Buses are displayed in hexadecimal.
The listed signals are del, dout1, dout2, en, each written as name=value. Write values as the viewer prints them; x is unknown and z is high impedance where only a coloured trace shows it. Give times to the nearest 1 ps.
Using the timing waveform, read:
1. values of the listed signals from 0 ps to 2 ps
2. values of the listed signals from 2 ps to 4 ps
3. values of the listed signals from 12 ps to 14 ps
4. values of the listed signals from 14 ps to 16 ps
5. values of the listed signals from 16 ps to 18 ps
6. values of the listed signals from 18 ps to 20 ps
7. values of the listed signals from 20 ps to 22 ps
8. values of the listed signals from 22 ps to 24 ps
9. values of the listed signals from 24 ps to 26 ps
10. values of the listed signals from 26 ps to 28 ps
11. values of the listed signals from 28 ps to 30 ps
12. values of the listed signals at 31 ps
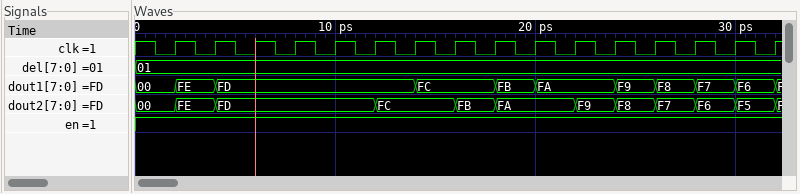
del=01, dout1=00, dout2=00, en=1
del=01, dout1=FE, dout2=FE, en=1
del=01, dout1=FD, dout2=FC, en=1
del=01, dout1=FC, dout2=FC, en=1
del=01, dout1=FC, dout2=FB, en=1
del=01, dout1=FB, dout2=FA, en=1
del=01, dout1=FA, dout2=FA, en=1
del=01, dout1=FA, dout2=F9, en=1
del=01, dout1=F9, dout2=F8, en=1
del=01, dout1=F8, dout2=F7, en=1
del=01, dout1=F7, dout2=F6, en=1
del=01, dout1=F6, dout2=F5, en=1
